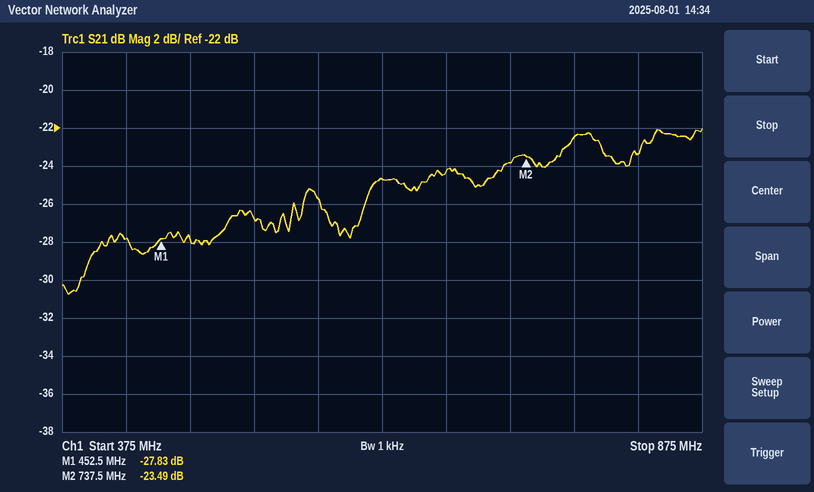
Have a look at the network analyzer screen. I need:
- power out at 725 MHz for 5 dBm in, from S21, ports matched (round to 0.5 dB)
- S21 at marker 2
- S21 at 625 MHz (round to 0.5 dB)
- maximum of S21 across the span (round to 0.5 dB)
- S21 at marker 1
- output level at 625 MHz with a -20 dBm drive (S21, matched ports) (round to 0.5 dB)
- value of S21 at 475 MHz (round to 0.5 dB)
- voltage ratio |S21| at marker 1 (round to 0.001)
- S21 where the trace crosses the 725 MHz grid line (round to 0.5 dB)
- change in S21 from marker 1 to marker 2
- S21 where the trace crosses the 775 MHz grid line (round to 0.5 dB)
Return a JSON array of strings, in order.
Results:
["-19.0 dBm", "-23.49 dB", "-24.5 dB", "-22.0 dB", "-27.83 dB", "-44.5 dBm", "-28.0 dB", "0.041", "-24.0 dB", "4.34 dB", "-22.5 dB"]
